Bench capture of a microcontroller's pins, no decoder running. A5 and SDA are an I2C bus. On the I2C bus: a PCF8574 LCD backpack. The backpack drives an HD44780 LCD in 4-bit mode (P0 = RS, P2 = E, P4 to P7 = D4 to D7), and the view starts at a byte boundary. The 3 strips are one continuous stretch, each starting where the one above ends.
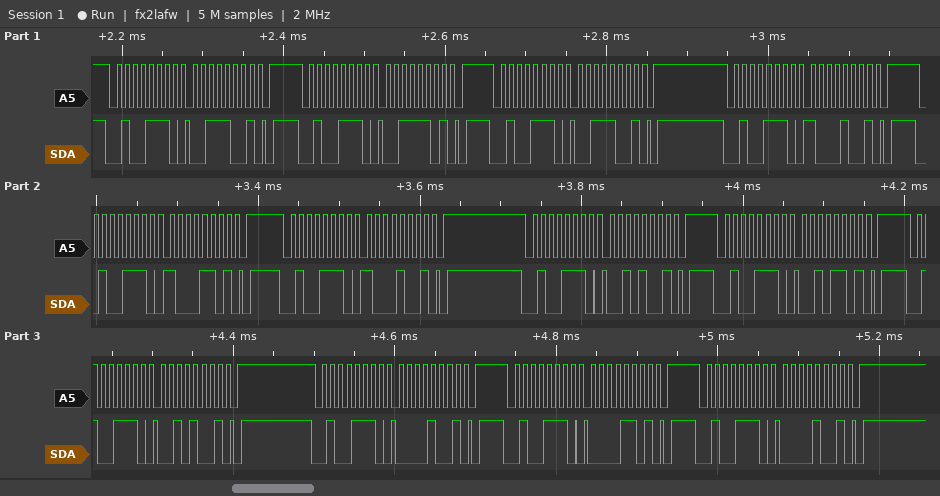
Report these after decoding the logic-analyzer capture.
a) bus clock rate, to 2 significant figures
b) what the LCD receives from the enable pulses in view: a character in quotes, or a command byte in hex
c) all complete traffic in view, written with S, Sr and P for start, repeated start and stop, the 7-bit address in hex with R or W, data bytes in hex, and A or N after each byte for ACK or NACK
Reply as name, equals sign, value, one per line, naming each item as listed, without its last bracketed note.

bus clock rate, to 2 significant figures = 100 kHz
what the LCD receives from the enable pulses in view: a character in quotes, or a command byte in hex = '8' ' '
all complete traffic in view, written with S, Sr and P for start, repeated start and stop, the 7-bit address in hex with R or W, data bytes in hex, and A or N after each byte for ACK or NACK = S 27W A 39 A P S 27W A 3D A P S 27W A 39 A P S 27W A 89 A P S 27W A 8D A P S 27W A 89 A P S 27W A 29 A P S 27W A 2D A P S 27W A 29 A P S 27W A 09 A P S 27W A 0D A P S 27W A 09 A P
